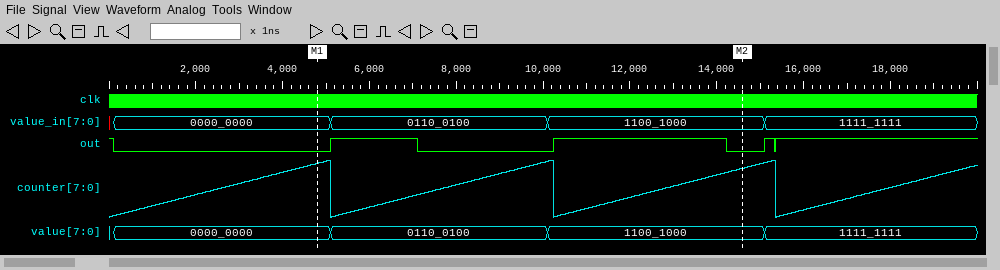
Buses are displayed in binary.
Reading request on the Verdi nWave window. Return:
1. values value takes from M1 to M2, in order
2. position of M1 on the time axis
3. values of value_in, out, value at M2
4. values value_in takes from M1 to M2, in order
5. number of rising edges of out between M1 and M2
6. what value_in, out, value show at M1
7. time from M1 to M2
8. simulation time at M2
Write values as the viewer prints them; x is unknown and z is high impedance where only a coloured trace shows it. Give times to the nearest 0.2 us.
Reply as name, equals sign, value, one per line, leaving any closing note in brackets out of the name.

values value takes from M1 to M2, in order = 0000_0000, 0110_0100, 1100_1000
position of M1 on the time axis = 4.8 us
values of value_in, out, value at M2 = value_in=1100_1000, out=0, value=1100_1000
values value_in takes from M1 to M2, in order = 0000_0000, 0110_0100, 1100_1000
number of rising edges of out between M1 and M2 = 2
what value_in, out, value show at M1 = value_in=0000_0000, out=0, value=0000_0000
time from M1 to M2 = 9.8 us
simulation time at M2 = 14.6 us
